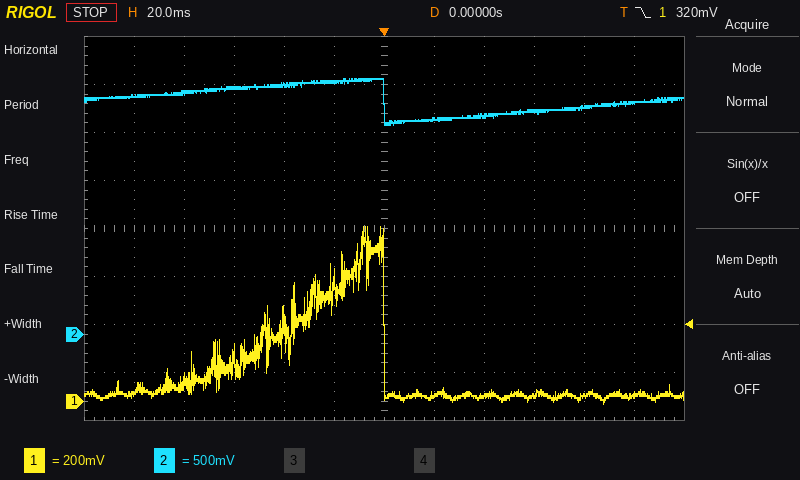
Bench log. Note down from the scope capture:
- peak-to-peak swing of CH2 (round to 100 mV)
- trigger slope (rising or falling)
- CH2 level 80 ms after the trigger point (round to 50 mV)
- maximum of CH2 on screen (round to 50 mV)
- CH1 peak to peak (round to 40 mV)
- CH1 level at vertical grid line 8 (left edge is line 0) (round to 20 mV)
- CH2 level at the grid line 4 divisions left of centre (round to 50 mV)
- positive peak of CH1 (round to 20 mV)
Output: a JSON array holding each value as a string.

["500 mV", "falling", "2.35 V", "2.65 V", "720 mV", "20 mV", "2.50 V", "720 mV"]
